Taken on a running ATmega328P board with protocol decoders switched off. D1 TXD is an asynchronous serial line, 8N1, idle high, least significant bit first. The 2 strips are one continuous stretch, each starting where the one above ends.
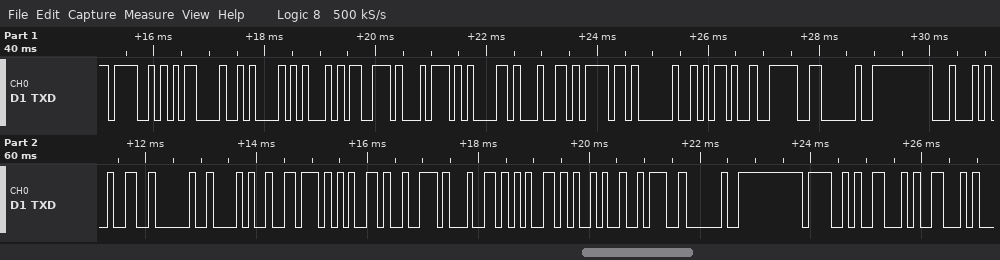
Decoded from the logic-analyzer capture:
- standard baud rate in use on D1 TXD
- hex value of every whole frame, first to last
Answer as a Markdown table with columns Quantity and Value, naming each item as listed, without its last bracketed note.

| Quantity | Value |
|---|---|
| standard baud rate in use on D1 TXD | 9600 baud |
| hex value of every whole frame, first to last | 0x4F 0x0D 0x0A 0x45 0x73 0x74 0x61 0x64 0x6F 0x20 0x2D 0x3E 0x20 0x44 0x32 0x20 0x28 0x76 0x65 0x72 0x64 0x65 0x29 0x3A 0x20 0x4F 0x46 0x46 |
